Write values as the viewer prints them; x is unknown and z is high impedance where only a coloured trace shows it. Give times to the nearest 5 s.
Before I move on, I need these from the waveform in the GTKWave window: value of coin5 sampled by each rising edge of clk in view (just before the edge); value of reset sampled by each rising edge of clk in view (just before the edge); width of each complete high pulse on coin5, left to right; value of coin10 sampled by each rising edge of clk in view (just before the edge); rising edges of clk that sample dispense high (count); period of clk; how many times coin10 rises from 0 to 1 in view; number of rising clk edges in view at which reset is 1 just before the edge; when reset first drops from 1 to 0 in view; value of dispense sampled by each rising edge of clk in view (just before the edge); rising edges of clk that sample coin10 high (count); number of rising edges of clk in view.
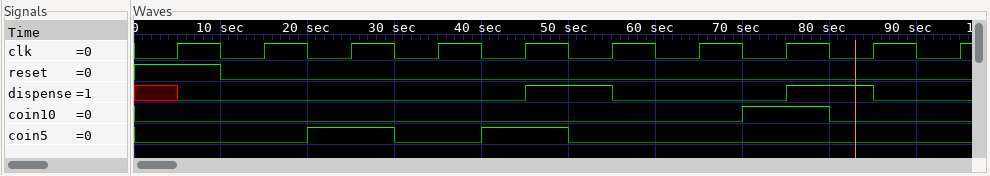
0 0 1 0 1 0 0 0 0 0
1 0 0 0 0 0 0 0 0 0
10 s, 10 s
0 0 0 0 0 0 0 1 0 0
2
10 s
1
1
10 s
x 0 0 0 0 1 0 0 1 0
1
10
